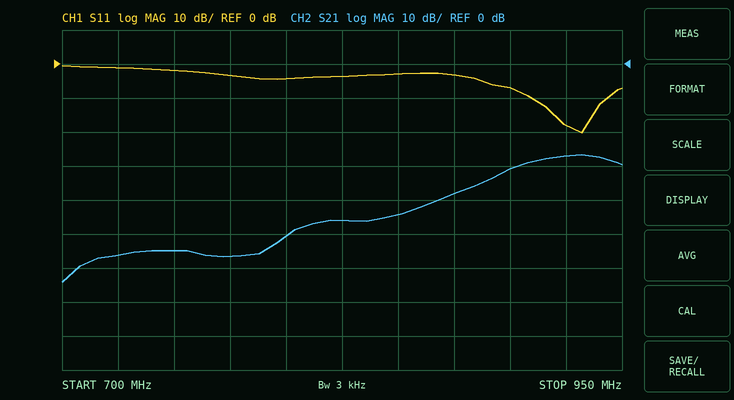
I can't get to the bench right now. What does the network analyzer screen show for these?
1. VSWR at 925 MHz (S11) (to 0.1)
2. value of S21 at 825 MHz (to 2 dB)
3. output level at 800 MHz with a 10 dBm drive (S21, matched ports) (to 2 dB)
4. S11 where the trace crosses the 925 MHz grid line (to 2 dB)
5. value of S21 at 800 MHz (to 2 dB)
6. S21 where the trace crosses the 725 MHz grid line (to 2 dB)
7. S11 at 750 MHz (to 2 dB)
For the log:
1.3
-46 dB
-40 dBm
-18 dB
-50 dB
-56 dB
-2 dB
